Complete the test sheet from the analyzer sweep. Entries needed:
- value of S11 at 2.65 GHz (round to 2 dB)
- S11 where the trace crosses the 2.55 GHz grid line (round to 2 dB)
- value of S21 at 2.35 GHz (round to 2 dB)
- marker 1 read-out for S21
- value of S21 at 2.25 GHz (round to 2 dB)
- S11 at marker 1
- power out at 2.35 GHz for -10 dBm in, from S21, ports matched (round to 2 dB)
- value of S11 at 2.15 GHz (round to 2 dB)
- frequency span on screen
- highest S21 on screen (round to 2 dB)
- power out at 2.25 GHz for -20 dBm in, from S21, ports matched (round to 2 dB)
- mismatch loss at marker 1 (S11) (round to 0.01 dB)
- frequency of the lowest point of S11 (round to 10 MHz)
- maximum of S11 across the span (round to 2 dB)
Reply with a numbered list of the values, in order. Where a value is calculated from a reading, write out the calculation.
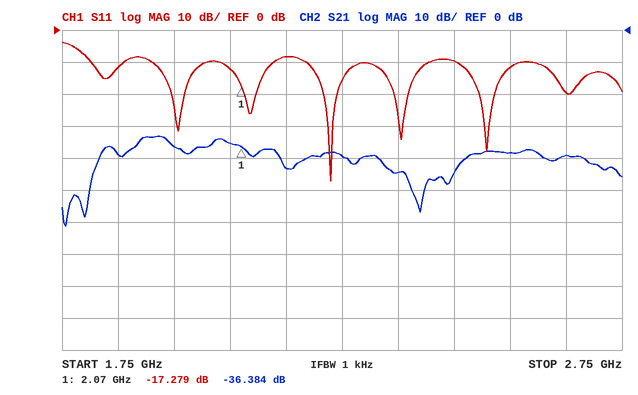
1. -20 dB
2. -12 dB
3. -44 dB
4. -36.384 dB
5. -40 dB
6. -17.279 dB
7. -10 dBm + (-44 dB) = -54 dBm
8. -8 dB
9. 1 GHz
10. -34 dB
11. -20 dBm + (-40 dB) = -60 dBm
12. −10 log10(1 − 10^(-17.279/10)) ≈ 0.08 dB
13. 2.23 GHz
14. -4 dB
